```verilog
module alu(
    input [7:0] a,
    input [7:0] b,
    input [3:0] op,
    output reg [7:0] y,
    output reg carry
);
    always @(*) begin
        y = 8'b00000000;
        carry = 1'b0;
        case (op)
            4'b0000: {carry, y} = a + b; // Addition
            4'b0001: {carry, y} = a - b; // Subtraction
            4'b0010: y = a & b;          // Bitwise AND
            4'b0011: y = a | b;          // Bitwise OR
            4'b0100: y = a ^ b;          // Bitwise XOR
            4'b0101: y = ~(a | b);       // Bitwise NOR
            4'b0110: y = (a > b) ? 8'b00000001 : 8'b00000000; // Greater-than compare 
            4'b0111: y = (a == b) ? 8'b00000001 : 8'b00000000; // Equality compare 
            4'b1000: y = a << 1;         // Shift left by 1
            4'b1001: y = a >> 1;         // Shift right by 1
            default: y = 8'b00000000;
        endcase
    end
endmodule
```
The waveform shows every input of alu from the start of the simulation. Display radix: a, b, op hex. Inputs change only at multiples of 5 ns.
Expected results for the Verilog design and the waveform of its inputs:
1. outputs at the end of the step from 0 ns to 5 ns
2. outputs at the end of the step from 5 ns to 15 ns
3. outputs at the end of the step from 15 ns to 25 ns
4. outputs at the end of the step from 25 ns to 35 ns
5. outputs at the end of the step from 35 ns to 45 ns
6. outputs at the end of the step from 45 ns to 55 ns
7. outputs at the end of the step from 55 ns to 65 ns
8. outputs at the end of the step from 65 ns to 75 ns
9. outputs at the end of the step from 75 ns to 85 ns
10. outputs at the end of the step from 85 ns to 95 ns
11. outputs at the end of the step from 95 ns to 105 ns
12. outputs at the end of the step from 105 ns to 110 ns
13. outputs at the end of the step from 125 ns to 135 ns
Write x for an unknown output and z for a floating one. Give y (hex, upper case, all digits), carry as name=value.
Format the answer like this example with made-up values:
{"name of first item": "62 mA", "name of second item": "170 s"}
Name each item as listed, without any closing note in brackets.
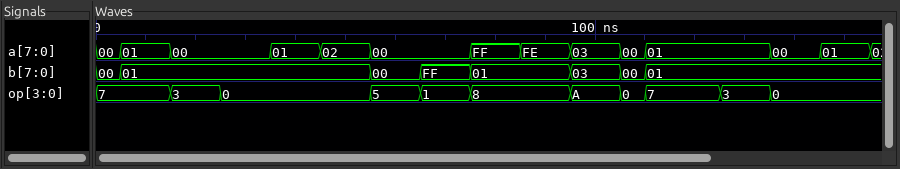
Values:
{"outputs at the end of the step from 0 ns to 5 ns": "y=01, carry=0", "outputs at the end of the step from 5 ns to 15 ns": "y=01, carry=0", "outputs at the end of the step from 15 ns to 25 ns": "y=01, carry=0", "outputs at the end of the step from 25 ns to 35 ns": "y=01, carry=0", "outputs at the end of the step from 35 ns to 45 ns": "y=02, carry=0", "outputs at the end of the step from 45 ns to 55 ns": "y=03, carry=0", "outputs at the end of the step from 55 ns to 65 ns": "y=FF, carry=0", "outputs at the end of the step from 65 ns to 75 ns": "y=01, carry=1", "outputs at the end of the step from 75 ns to 85 ns": "y=FE, carry=0", "outputs at the end of the step from 85 ns to 95 ns": "y=FC, carry=0", "outputs at the end of the step from 95 ns to 105 ns": "y=00, carry=0", "outputs at the end of the step from 105 ns to 110 ns": "y=00, carry=0", "outputs at the end of the step from 125 ns to 135 ns": "y=01, carry=0"}
